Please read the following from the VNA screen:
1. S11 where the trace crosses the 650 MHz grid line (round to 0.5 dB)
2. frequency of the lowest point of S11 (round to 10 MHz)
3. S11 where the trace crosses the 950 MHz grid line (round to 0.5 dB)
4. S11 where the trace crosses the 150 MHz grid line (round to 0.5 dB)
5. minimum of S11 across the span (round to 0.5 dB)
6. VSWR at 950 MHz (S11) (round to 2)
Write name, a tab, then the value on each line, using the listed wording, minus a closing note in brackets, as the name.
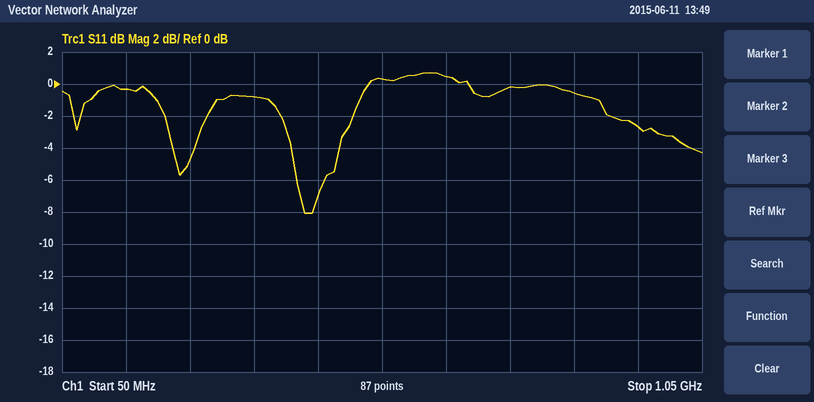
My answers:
S11 where the trace crosses the 650 MHz grid line	0.5 dB
frequency of the lowest point of S11	430 MHz
S11 where the trace crosses the 950 MHz grid line	-2.5 dB
S11 where the trace crosses the 150 MHz grid line	-0.5 dB
minimum of S11 across the span	-8.0 dB
VSWR at 950 MHz (S11)	6
